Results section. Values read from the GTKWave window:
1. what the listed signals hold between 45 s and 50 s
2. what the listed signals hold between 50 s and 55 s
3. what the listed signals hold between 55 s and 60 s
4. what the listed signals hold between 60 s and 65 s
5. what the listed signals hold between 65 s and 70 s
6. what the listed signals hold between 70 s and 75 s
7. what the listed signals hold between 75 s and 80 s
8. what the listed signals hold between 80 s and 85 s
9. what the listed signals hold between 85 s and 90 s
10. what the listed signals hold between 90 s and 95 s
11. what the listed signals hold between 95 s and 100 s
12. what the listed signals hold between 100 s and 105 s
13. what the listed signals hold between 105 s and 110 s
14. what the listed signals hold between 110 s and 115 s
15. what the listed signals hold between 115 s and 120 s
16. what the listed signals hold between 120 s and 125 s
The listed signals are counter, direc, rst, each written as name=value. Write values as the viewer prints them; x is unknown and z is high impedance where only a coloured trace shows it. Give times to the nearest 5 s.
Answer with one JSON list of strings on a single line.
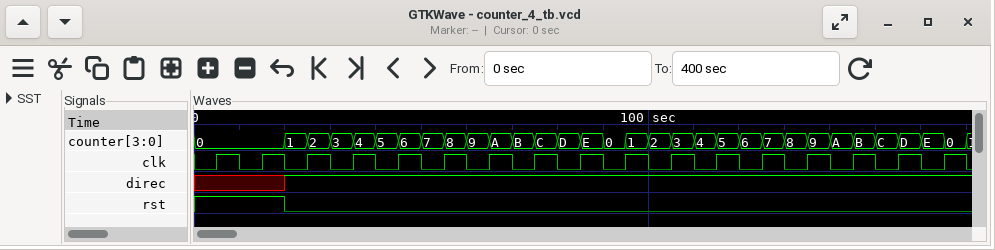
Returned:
["counter=6, direc=1, rst=0", "counter=7, direc=1, rst=0", "counter=8, direc=1, rst=0", "counter=9, direc=1, rst=0", "counter=A, direc=1, rst=0", "counter=B, direc=1, rst=0", "counter=C, direc=1, rst=0", "counter=D, direc=1, rst=0", "counter=E, direc=1, rst=0", "counter=0, direc=1, rst=0", "counter=1, direc=1, rst=0", "counter=2, direc=1, rst=0", "counter=3, direc=1, rst=0", "counter=4, direc=1, rst=0", "counter=5, direc=1, rst=0", "counter=6, direc=1, rst=0"]
